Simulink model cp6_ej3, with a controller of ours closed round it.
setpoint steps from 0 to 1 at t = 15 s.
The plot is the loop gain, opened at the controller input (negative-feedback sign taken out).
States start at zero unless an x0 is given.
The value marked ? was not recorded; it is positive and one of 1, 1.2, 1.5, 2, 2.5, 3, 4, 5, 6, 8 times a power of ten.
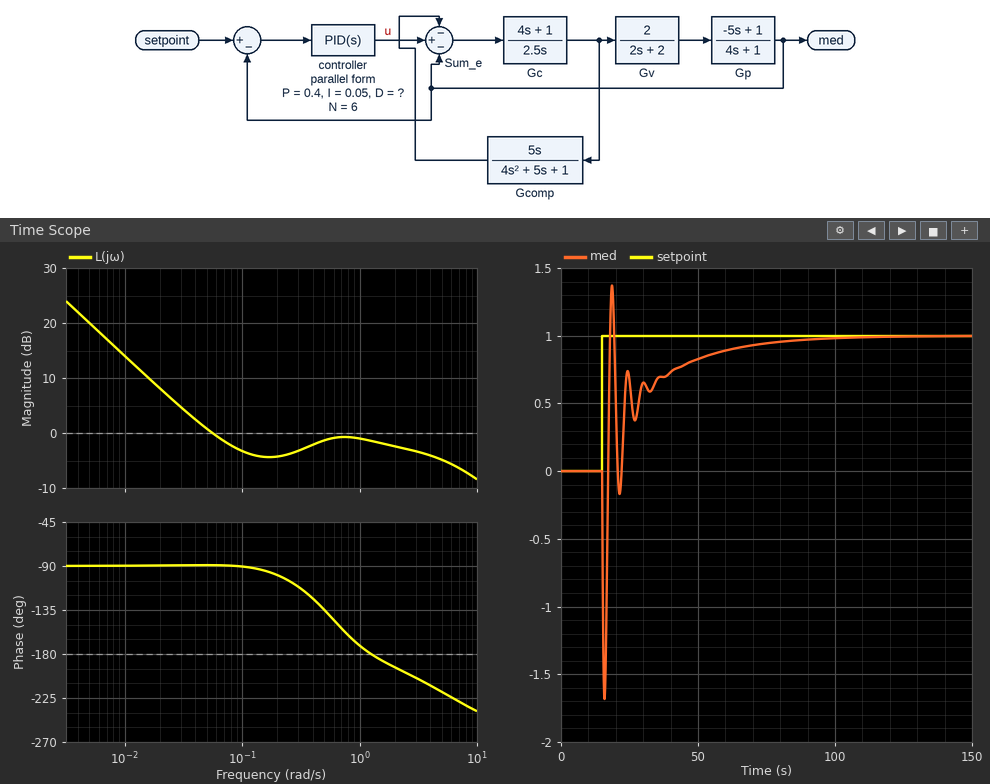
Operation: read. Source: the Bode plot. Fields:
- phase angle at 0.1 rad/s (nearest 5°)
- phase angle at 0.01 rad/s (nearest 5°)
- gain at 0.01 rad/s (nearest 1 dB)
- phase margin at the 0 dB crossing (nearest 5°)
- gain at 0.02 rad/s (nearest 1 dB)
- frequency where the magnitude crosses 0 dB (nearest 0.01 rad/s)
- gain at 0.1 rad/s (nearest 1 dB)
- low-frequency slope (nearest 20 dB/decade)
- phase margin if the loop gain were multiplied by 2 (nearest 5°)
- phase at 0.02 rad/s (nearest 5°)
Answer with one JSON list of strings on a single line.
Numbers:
["-90°", "-90°", "14 dB", "90°", "8 dB", "0.06 rad/s", "-3 dB", "-20 dB/decade", "-45°", "-90°"]
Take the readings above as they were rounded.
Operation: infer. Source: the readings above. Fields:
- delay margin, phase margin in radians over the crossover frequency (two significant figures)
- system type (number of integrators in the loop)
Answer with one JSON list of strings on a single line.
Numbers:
["26 s", "1"]
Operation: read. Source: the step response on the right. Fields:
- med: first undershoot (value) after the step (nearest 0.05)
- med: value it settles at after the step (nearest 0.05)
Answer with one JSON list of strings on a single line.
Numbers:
["-0.15", "1.00"]
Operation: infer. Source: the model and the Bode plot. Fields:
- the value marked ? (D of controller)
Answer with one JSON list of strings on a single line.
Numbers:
["0.3"]
